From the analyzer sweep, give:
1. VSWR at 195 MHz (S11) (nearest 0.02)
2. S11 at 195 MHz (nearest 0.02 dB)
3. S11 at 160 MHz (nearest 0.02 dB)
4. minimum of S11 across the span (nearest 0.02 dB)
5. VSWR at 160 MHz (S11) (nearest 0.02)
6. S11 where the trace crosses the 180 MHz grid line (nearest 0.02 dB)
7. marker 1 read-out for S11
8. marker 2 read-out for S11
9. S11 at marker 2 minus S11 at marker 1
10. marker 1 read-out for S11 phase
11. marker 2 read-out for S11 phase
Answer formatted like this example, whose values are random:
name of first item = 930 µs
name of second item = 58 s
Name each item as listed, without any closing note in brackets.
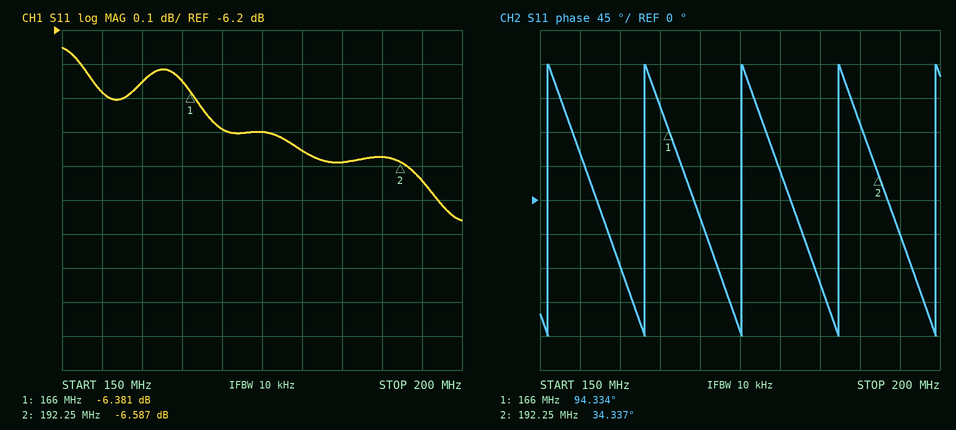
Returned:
VSWR at 195 MHz (S11) = 2.74
S11 at 195 MHz = -6.64 dB
S11 at 160 MHz = -6.36 dB
minimum of S11 across the span = -6.76 dB
VSWR at 160 MHz (S11) = 2.86
S11 where the trace crosses the 180 MHz grid line = -6.56 dB
marker 1 read-out for S11 = -6.381 dB
marker 2 read-out for S11 = -6.587 dB
S11 at marker 2 minus S11 at marker 1 = -0.206 dB
marker 1 read-out for S11 phase = 94.334°
marker 2 read-out for S11 phase = 34.337°
